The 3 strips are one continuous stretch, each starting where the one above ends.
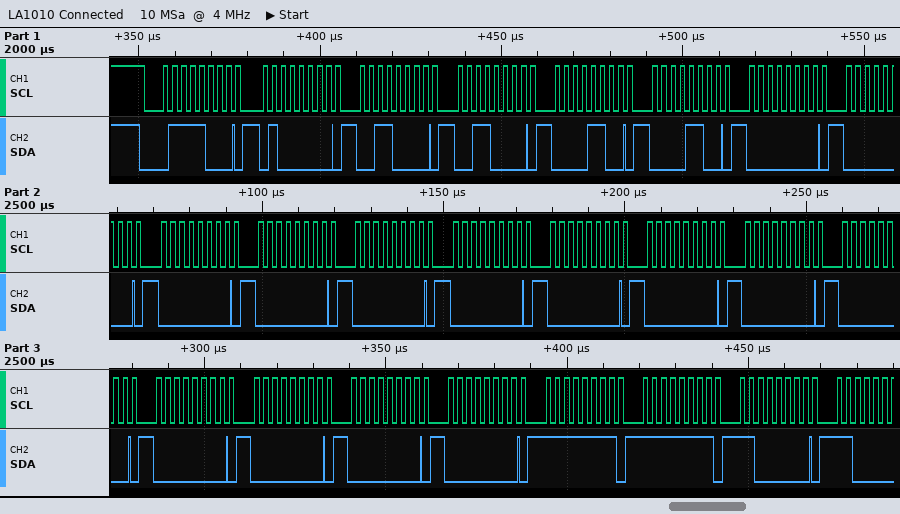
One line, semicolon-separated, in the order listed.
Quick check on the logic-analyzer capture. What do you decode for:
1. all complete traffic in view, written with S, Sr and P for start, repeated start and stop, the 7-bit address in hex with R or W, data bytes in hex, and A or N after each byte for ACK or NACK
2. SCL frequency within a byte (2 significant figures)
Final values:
S 3CW A 40 A 30 A 30 A 0C A 0C A 00 A 00 A 00 A 00 A 00 A 00 A 00 A 00 A 00 A 00 A 00 A 00 A 00 A 00 A FF A FF A C0 A; 400 kHz
